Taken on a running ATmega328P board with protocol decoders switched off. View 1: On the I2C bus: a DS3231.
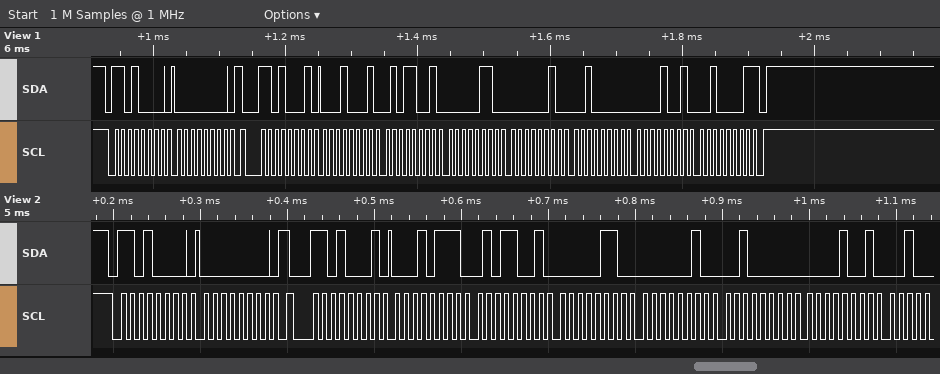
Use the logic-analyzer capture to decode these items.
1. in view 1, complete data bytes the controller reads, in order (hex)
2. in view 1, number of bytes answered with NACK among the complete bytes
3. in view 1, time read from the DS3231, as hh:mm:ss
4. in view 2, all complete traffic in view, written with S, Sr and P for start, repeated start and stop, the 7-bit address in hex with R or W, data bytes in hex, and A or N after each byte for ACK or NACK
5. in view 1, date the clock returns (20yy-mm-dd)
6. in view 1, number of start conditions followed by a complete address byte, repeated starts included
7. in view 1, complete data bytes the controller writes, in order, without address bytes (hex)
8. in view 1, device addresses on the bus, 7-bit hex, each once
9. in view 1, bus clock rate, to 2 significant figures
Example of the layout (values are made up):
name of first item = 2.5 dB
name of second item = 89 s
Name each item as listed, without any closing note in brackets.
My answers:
in view 1, complete data bytes the controller reads, in order = 11 59 06 02 20 09 21
in view 1, number of bytes answered with NACK among the complete bytes = 1
in view 1, time read from the DS3231, as hh:mm:ss = 06:59:11
in view 2, all complete traffic in view, written with S, Sr and P for start, repeated start and stop, the 7-bit address in hex with R or W, data bytes in hex, and A or N after each byte for ACK or NACK = S 68W A 00 A Sr 68R A 17 A 59 A 06 A 02 A 20 A 09 A
in view 1, date the clock returns = 2021-09-20
in view 1, number of start conditions followed by a complete address byte, repeated starts included = 2
in view 1, complete data bytes the controller writes, in order, without address bytes = 00
in view 1, device addresses on the bus, 7-bit hex, each once = 0x68
in view 1, bus clock rate, to 2 significant figures = 100 kHz
